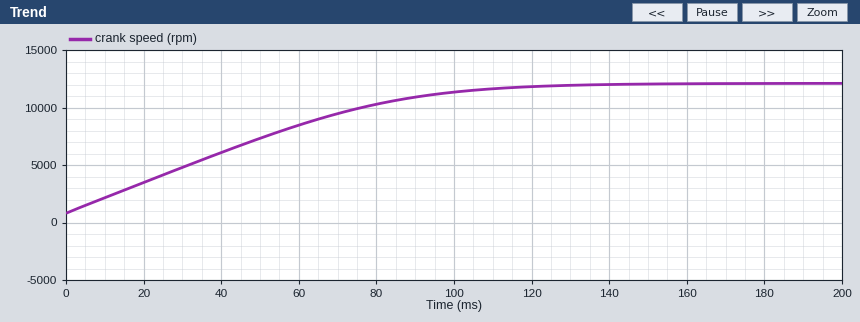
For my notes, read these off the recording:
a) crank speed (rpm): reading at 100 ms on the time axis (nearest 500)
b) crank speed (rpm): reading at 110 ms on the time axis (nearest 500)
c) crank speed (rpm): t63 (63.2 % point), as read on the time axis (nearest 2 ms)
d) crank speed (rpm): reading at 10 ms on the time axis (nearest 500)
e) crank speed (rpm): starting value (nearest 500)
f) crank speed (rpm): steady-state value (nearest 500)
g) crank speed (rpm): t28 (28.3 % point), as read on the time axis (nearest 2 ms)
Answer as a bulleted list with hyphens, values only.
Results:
- 11500
- 11500
- 56 ms
- 2000
- 1000
- 12000
- 24 ms
